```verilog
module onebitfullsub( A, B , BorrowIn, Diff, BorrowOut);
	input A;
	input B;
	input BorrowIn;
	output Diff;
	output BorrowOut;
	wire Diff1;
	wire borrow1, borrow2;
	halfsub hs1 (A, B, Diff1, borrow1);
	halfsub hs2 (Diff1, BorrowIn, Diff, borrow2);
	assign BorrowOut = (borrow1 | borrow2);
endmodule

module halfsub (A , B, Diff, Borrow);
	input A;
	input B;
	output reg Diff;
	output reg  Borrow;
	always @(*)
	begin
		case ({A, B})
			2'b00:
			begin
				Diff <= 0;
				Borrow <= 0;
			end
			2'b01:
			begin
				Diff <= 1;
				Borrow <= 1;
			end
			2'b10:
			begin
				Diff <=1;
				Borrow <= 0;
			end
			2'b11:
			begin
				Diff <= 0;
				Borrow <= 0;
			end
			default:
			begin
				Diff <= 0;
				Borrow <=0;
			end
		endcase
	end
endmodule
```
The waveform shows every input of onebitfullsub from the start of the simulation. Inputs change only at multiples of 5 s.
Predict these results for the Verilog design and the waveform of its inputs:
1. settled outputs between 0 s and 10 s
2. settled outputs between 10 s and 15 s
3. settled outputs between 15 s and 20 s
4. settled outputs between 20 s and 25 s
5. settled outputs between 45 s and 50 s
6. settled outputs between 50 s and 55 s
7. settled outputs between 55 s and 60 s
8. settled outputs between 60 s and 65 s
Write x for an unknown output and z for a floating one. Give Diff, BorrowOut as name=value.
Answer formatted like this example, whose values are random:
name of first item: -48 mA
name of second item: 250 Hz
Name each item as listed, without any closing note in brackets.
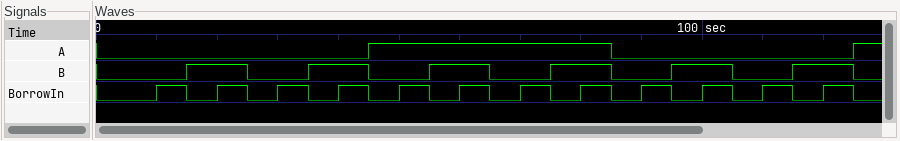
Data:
settled outputs between 0 s and 10 s: Diff=0, BorrowOut=0
settled outputs between 10 s and 15 s: Diff=1, BorrowOut=1
settled outputs between 15 s and 20 s: Diff=1, BorrowOut=1
settled outputs between 20 s and 25 s: Diff=0, BorrowOut=1
settled outputs between 45 s and 50 s: Diff=1, BorrowOut=0
settled outputs between 50 s and 55 s: Diff=0, BorrowOut=0
settled outputs between 55 s and 60 s: Diff=0, BorrowOut=0
settled outputs between 60 s and 65 s: Diff=1, BorrowOut=1
